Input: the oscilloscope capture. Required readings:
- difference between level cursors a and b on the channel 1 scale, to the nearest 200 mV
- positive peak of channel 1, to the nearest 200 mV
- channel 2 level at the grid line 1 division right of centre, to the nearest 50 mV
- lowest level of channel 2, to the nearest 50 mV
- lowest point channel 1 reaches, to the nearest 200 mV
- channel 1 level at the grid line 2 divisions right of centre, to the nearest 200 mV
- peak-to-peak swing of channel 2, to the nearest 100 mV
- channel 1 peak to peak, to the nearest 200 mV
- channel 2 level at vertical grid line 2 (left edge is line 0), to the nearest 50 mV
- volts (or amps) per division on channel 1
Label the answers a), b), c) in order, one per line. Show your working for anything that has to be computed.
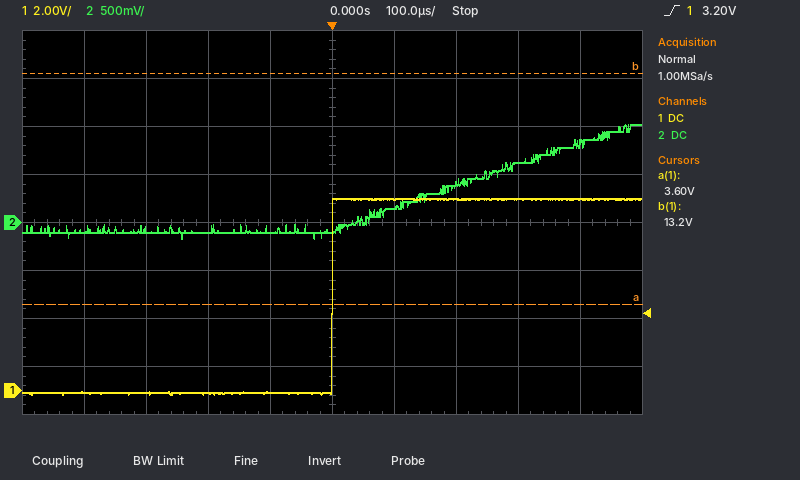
a) 9.6 V
b) 8.0 V
c) 150 mV
d) -150 mV
e) -200 mV
f) 8.0 V
g) 1.20 V
h) 8.0 V − (-200 mV) = 8.2 V
i) -50 mV
j) 2 V
